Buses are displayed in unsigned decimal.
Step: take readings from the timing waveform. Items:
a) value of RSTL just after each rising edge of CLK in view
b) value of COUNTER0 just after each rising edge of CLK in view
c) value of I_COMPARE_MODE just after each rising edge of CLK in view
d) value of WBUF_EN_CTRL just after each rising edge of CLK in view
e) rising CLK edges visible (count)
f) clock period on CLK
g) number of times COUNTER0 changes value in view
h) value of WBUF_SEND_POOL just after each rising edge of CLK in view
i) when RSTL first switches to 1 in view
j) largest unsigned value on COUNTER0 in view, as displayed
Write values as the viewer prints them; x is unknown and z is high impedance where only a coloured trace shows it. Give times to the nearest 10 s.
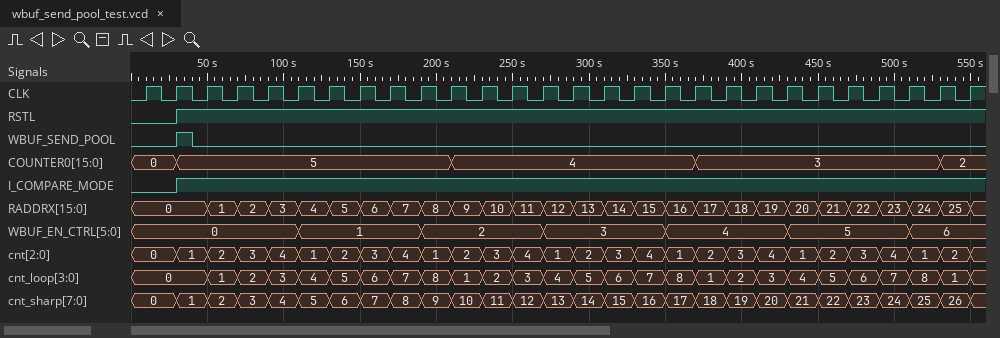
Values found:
0 1 1 1 1 1 1 1 1 1 1 1 1 1 1 1 1 1 1 1 1 1 1 1 1 1 1 1
0, 5, 5, 5, 5, 5, 5, 5, 5, 5, 4, 4, 4, 4, 4, 4, 4, 4, 3, 3, 3, 3, 3, 3, 3, 3, 2, 2
0 1 1 1 1 1 1 1 1 1 1 1 1 1 1 1 1 1 1 1 1 1 1 1 1 1 1 1
0, 0, 0, 0, 0, 1, 1, 1, 1, 2, 2, 2, 2, 3, 3, 3, 3, 4, 4, 4, 4, 5, 5, 5, 5, 6, 6, 6
28
20 s
4
0 1 0 0 0 0 0 0 0 0 0 0 0 0 0 0 0 0 0 0 0 0 0 0 0 0 0 0
30 s
5
